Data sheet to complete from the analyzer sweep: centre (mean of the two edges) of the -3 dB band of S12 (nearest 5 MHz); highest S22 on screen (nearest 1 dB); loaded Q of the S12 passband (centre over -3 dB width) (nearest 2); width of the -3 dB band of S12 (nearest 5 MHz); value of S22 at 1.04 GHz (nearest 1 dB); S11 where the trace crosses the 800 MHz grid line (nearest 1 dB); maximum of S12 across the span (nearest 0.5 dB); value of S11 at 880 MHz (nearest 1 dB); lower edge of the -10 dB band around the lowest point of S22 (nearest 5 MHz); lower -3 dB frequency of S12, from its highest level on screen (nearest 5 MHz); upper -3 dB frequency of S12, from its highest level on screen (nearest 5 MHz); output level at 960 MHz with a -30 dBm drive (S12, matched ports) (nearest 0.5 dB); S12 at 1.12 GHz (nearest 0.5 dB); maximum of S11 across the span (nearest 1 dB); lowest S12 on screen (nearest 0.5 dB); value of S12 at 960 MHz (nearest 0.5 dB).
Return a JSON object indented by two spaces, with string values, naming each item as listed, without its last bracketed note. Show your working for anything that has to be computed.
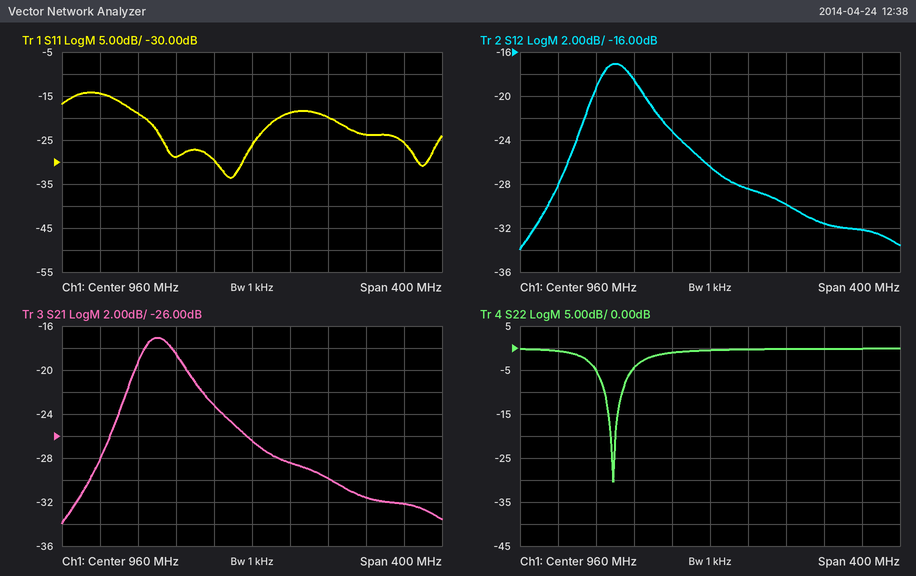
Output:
{
  "centre (mean of the two edges) of the -3 dB band of S12": "865 MHz",
  "highest S22 on screen": "0 dB",
  "loaded Q of the S12 passband (centre over -3 dB width)": "862.5 MHz / 55 MHz ≈ 16",
  "width of the -3 dB band of S12": "890 MHz − 835 MHz = 55 MHz",
  "value of S22 at 1.04 GHz": "0 dB",
  "S11 where the trace crosses the 800 MHz grid line": "-14 dB",
  "maximum of S12 across the span": "-17.0 dB",
  "value of S11 at 880 MHz": "-29 dB",
  "lower edge of the -10 dB band around the lowest point of S22": "850 MHz",
  "lower -3 dB frequency of S12, from its highest level on screen": "835 MHz",
  "upper -3 dB frequency of S12, from its highest level on screen": "890 MHz",
  "output level at 960 MHz with a -30 dBm drive (S12, matched ports)": "-30 dBm + (-26.5 dB) = -56.5 dBm",
  "S12 at 1.12 GHz": "-32.0 dB",
  "maximum of S11 across the span": "-14 dB",
  "lowest S12 on screen": "-34.0 dB",
  "value of S12 at 960 MHz": "-26.5 dB"
}
